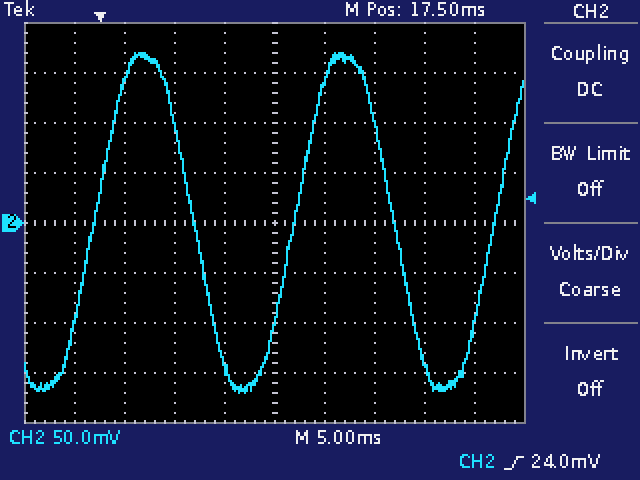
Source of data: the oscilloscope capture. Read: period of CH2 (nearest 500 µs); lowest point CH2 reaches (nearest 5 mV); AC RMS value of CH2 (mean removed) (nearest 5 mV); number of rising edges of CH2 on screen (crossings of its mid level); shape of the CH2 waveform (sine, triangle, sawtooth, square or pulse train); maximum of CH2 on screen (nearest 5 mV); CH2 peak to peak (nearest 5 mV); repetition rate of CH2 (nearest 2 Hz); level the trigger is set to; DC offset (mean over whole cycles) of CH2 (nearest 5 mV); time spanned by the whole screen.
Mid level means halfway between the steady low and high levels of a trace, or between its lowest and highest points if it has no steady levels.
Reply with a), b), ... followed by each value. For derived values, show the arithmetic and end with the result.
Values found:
a) 20.0 ms
b) -170 mV
c) 340 mV / (2√2) ≈ 120 mV
d) 3
e) sine
f) 170 mV
g) 170 mV − (-170 mV) = 340 mV
h) 1 / 20.0 ms ≈ 50 Hz
i) 24.0 mV
j) (170 mV + (-170 mV)) / 2 ≈ 0 mV
k) 50 ms
